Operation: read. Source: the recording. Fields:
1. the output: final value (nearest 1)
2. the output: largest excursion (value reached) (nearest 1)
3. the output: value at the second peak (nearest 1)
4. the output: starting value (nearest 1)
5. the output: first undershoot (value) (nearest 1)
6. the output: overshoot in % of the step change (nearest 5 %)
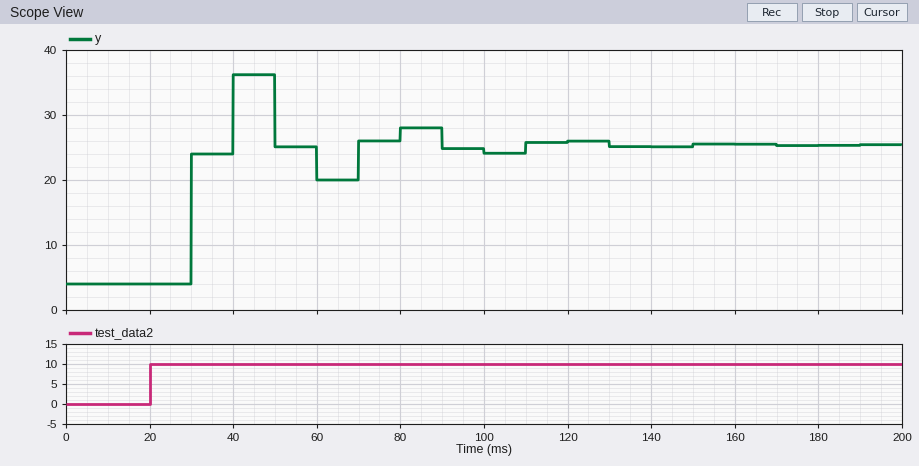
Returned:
25
36
28
4
20
50 %
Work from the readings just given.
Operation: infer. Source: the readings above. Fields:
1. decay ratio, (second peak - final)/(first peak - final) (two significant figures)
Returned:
0.27
